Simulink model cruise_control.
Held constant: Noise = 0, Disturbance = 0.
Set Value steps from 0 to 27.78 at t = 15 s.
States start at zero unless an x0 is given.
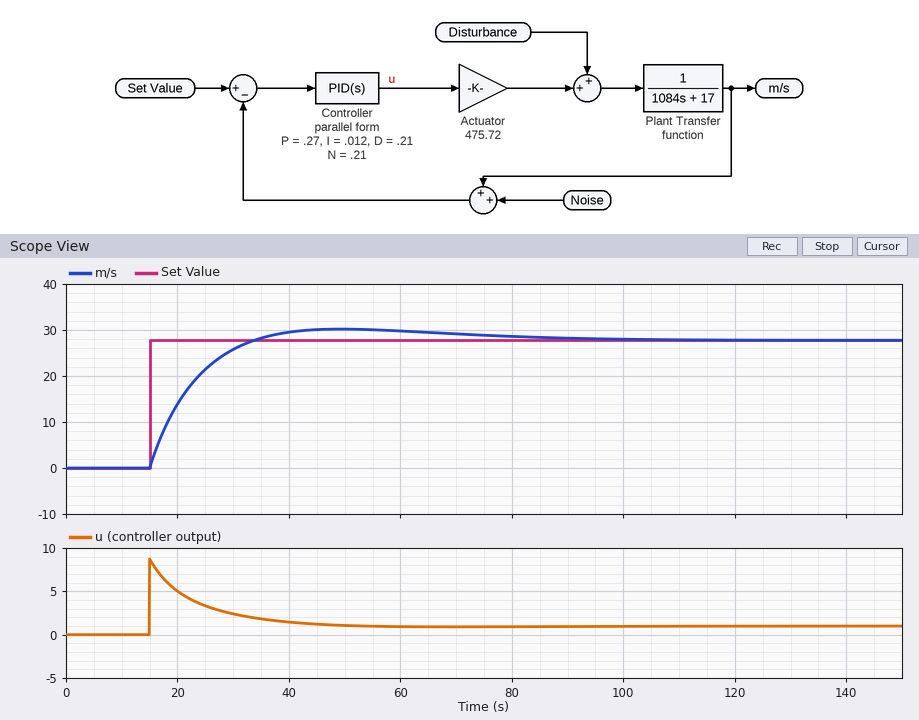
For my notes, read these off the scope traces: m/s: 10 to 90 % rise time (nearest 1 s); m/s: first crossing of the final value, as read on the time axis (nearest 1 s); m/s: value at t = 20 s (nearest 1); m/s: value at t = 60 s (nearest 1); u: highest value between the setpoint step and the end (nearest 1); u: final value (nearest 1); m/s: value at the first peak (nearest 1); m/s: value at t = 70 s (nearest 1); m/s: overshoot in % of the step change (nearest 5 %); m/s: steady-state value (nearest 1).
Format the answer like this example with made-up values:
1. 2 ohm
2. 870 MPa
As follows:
1. 13 s
2. 34 s
3. 14
4. 30
5. 9
6. 1
7. 30
8. 29
9. 10 %
10. 28
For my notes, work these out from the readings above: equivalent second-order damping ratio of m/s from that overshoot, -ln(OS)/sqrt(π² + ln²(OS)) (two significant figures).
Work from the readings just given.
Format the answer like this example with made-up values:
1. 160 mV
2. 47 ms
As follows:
1. 0.59
